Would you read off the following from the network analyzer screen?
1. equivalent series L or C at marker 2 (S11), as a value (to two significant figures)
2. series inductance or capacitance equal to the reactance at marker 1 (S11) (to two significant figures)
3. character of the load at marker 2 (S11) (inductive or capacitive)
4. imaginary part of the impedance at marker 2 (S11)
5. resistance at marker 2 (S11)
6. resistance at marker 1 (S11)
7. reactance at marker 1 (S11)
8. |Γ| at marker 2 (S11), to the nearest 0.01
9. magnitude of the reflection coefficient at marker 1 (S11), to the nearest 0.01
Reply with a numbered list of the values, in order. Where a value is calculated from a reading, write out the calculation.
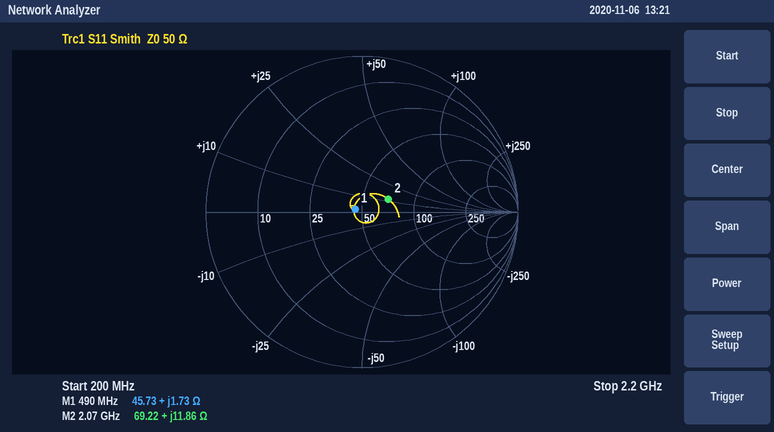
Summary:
1. L = 11.86 Ω/(2π × 2.07 GHz) ≈ 912 pH, so 910 pH to two significant figures
2. L = 1.73 Ω/(2π × 490 MHz) ≈ 562 pH, so 560 pH to two significant figures
3. inductive
4. +11.86 Ω
5. 69.22 Ω
6. 45.73 Ω
7. +1.73 Ω
8. 0.19
9. 0.05
